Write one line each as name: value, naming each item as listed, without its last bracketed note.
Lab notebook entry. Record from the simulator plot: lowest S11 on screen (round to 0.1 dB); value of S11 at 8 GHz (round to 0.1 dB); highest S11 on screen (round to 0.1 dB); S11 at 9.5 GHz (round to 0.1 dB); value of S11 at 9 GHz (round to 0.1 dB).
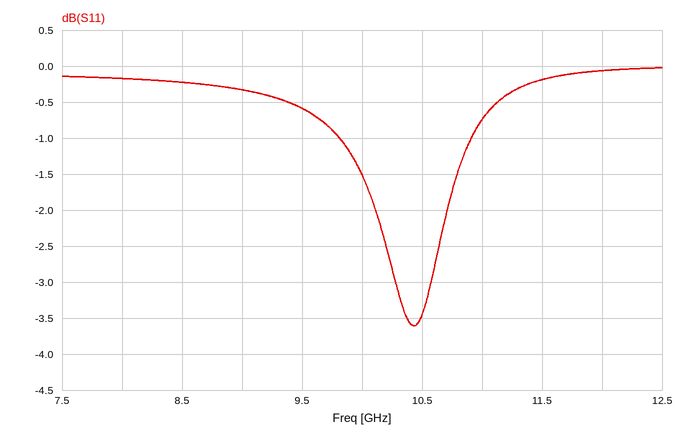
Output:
lowest S11 on screen: -3.6 dB
value of S11 at 8 GHz: -0.2 dB
highest S11 on screen: 0.0 dB
S11 at 9.5 GHz: -0.6 dB
value of S11 at 9 GHz: -0.3 dB
